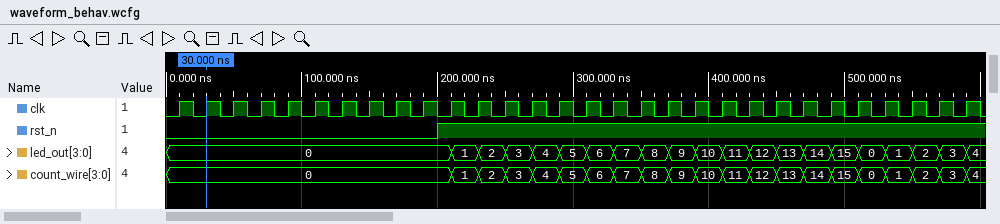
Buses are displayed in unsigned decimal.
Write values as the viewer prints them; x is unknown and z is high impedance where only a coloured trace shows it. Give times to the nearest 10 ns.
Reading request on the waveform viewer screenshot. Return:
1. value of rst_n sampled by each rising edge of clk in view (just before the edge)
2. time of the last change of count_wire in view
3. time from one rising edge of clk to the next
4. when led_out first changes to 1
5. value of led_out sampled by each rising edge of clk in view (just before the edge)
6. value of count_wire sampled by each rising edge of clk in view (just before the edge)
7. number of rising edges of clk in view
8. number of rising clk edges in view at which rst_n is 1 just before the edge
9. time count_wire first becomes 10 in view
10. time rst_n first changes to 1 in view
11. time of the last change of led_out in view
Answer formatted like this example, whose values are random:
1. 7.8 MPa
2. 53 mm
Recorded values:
1. 0 0 0 0 0 0 0 0 0 0 1 1 1 1 1 1 1 1 1 1 1 1 1 1 1 1 1 1 1 1
2. 590 ns
3. 20 ns
4. 210 ns
5. 0, 0, 0, 0, 0, 0, 0, 0, 0, 0, 0, 1, 2, 3, 4, 5, 6, 7, 8, 9, 10, 11, 12, 13, 14, 15, 0, 1, 2, 3
6. 0, 0, 0, 0, 0, 0, 0, 0, 0, 0, 0, 1, 2, 3, 4, 5, 6, 7, 8, 9, 10, 11, 12, 13, 14, 15, 0, 1, 2, 3
7. 30
8. 20
9. 390 ns
10. 200 ns
11. 590 ns
